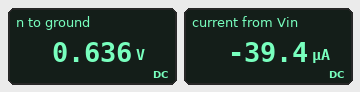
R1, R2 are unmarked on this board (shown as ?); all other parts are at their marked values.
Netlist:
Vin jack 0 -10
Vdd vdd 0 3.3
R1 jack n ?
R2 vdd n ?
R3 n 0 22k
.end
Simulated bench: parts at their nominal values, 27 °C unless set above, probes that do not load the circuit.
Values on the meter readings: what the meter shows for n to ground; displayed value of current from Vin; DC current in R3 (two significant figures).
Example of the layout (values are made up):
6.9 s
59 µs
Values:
0.636 V
-39.4 µA
29 µA
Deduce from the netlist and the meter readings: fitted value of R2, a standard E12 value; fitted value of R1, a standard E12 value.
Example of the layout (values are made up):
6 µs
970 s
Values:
39 kΩ
270 kΩ
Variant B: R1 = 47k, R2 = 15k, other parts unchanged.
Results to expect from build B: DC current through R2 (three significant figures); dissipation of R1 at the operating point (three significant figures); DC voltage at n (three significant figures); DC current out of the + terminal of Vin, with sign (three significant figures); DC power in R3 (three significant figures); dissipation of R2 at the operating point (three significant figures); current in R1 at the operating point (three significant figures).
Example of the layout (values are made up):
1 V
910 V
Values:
216 µA
2.15 mW
54.2 mV
-214 µA
134 nW
702 µW
214 µA
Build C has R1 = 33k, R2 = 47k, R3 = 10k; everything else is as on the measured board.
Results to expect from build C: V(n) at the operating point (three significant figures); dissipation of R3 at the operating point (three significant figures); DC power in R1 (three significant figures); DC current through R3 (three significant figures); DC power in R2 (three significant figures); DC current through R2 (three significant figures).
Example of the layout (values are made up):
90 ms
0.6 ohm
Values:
-1.54 V
236 µW
2.17 mW
154 µA
498 µW
103 µA
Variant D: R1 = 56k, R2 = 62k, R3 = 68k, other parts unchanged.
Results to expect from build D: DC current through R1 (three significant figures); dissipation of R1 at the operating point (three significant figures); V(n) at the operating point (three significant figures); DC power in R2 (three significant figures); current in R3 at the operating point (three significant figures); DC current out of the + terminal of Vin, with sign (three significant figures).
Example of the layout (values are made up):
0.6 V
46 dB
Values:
133 µA
985 µW
-2.57 V
557 µW
37.9 µA
-133 µA
